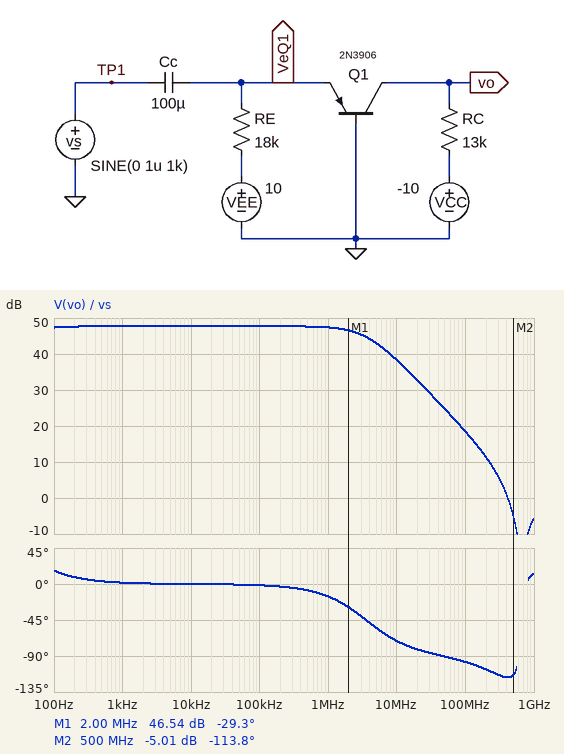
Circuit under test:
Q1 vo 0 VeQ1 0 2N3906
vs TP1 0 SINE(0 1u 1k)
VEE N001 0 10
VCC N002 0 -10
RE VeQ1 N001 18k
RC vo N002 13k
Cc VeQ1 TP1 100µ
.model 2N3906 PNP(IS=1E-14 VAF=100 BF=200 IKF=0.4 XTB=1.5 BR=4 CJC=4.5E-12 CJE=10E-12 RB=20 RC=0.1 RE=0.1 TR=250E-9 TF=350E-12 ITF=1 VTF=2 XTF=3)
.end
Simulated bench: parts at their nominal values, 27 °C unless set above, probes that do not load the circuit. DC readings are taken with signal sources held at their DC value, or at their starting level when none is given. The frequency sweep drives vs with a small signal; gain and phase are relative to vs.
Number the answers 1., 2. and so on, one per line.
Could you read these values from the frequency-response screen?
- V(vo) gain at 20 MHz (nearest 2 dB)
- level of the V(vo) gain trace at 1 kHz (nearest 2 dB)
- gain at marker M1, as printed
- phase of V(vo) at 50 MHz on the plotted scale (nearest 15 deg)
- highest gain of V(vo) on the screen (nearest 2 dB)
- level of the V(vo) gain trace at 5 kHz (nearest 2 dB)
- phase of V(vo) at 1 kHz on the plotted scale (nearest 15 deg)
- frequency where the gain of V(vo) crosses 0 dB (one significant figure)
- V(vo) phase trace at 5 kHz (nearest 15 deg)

1. 32 dB
2. 48 dB
3. 46.54 dB
4. -90 deg
5. 48 dB
6. 48 dB
7. 0 deg
8. 400 MHz
9. 0 deg
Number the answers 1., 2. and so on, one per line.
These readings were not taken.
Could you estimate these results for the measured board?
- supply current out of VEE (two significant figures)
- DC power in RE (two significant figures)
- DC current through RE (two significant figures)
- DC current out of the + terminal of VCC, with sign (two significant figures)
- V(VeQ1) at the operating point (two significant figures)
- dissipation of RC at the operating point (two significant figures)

1. 520 µA
2. 4.9 mW
3. 520 µA
4. -520 µA
5. 640 mV
6. 3.5 mW
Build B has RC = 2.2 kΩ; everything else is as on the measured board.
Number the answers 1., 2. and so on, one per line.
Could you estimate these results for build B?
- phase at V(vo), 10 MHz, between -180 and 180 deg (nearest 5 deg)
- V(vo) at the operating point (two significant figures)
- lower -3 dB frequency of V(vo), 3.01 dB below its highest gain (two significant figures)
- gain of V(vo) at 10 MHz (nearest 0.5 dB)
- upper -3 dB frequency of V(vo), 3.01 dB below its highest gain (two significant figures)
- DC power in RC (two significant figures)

1. -20 deg
2. -8.9 V
3. 32 Hz
4. 32.0 dB
5. 26 MHz
6. 590 µW
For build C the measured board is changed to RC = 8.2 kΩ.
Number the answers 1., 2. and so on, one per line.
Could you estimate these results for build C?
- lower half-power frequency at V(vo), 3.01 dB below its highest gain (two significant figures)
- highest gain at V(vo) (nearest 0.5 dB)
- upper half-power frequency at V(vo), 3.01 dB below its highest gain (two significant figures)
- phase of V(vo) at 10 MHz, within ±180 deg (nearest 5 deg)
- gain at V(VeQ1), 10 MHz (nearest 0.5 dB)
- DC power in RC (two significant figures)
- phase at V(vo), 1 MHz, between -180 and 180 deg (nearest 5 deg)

1. 31 Hz
2. 44.0 dB
3. 6.5 MHz
4. -60 deg
5. 0 dB
6. 2.2 mW
7. -10 deg
